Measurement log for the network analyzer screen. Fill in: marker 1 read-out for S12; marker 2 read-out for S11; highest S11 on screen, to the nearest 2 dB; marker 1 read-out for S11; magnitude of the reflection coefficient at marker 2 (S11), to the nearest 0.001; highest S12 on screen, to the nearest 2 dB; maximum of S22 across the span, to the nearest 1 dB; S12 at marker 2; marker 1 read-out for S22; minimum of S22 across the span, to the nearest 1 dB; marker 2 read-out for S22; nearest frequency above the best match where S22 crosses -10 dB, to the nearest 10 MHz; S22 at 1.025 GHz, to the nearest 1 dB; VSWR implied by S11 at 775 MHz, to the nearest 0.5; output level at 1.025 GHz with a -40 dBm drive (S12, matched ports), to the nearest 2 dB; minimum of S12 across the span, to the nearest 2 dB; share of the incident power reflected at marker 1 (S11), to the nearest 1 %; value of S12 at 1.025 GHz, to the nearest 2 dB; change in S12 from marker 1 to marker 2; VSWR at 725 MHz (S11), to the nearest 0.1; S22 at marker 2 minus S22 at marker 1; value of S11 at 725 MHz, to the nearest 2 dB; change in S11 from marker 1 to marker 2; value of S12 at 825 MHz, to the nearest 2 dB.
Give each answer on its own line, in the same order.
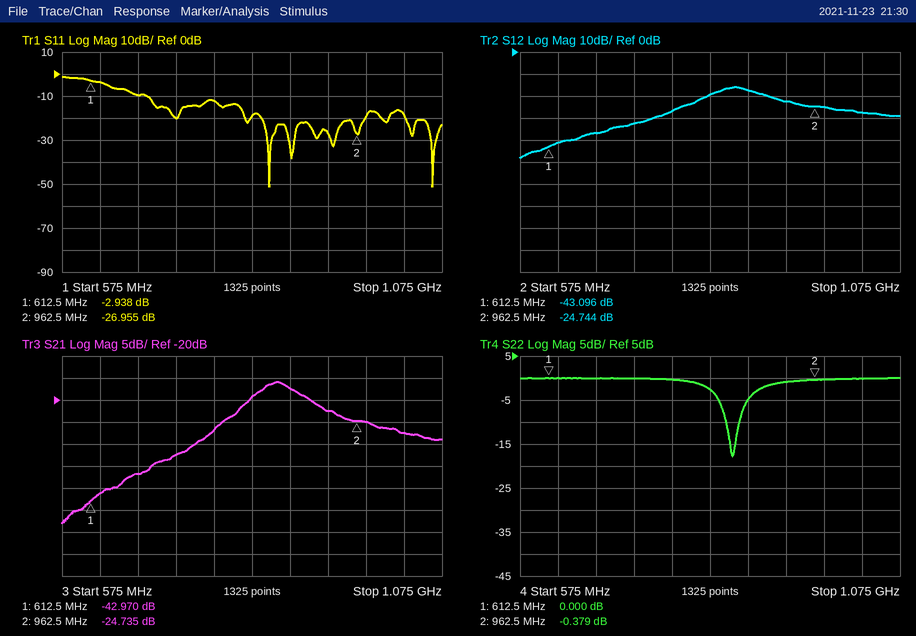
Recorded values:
-43.096 dB
-26.955 dB
-2 dB
-2.938 dB
0.045
-16 dB
0 dB
-24.744 dB
0.000 dB
-18 dB
-0.379 dB
860 MHz
0 dB
1.5
-68 dBm
-48 dB
51 %
-28 dB
18.352 dB
1.2
-0.379 dB
-20 dB
-24.017 dB
-20 dB
